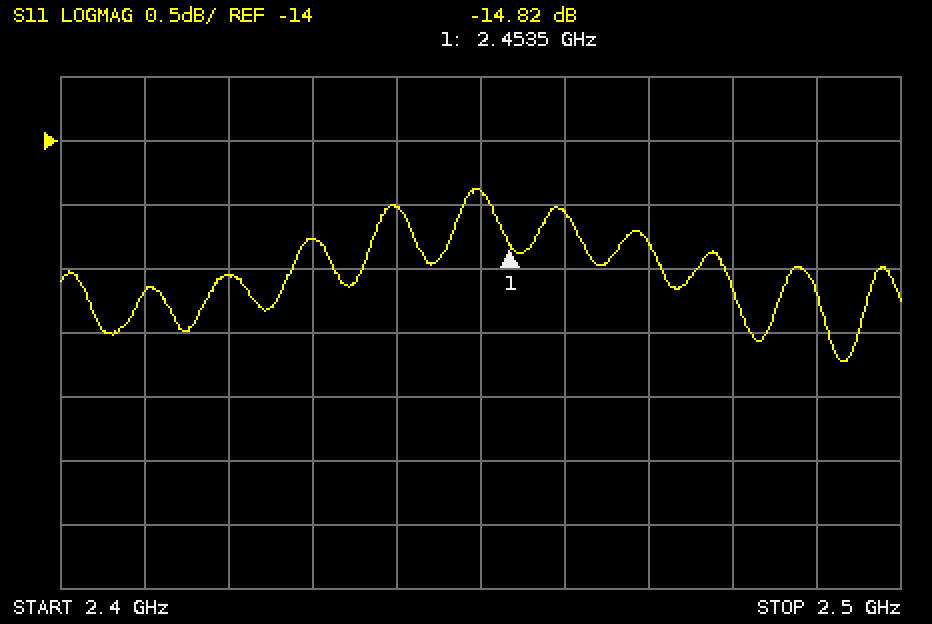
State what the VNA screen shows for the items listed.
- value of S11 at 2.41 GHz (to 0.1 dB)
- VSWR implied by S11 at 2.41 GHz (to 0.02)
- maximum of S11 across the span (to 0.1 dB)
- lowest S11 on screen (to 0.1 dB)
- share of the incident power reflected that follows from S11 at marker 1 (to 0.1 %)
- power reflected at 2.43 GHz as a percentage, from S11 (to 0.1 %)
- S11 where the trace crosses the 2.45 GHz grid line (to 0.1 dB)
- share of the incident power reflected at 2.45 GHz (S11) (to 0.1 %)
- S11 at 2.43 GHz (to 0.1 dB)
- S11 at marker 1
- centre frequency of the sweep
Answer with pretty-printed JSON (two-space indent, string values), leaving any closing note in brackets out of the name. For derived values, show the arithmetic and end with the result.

{
  "value of S11 at 2.41 GHz": "-15.2 dB",
  "VSWR implied by S11 at 2.41 GHz": "|Γ| = 10^(-15.2/20) = 0.1738; VSWR = (1 + 0.1738)/(1 − 0.1738) ≈ 1.42",
  "maximum of S11 across the span": "-14.4 dB",
  "lowest S11 on screen": "-15.7 dB",
  "share of the incident power reflected that follows from S11 at marker 1": "10^(-14.82/10) ≈ 3.3 %",
  "power reflected at 2.43 GHz as a percentage, from S11": "10^(-14.8/10) ≈ 3.3 %",
  "S11 where the trace crosses the 2.45 GHz grid line": "-14.4 dB",
  "share of the incident power reflected at 2.45 GHz (S11)": "10^(-14.4/10) ≈ 3.6 %",
  "S11 at 2.43 GHz": "-14.8 dB",
  "S11 at marker 1": "-14.82 dB",
  "centre frequency of the sweep": "2.45 GHz"
}
